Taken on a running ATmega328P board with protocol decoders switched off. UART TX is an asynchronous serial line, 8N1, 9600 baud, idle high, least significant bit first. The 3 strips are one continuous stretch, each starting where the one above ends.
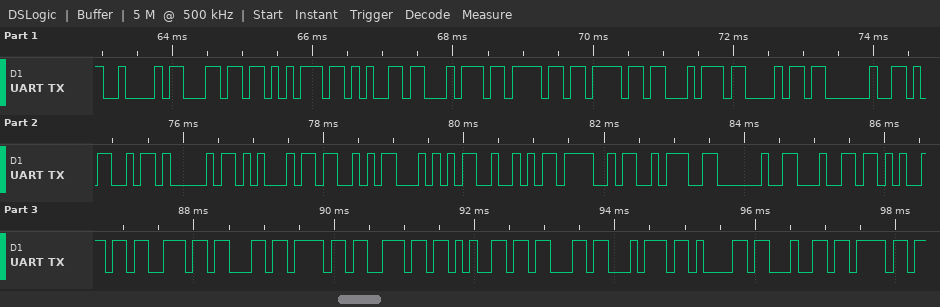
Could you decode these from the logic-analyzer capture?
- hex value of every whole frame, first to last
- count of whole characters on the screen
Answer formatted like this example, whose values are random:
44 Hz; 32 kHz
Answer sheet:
42 6C 75 65 74 6F 6F 74 68 20 4D 41 45 53 54 52 4F 3A 20 64 65 73 63 6F 6E 65 63 74 61 64 6F; 31
